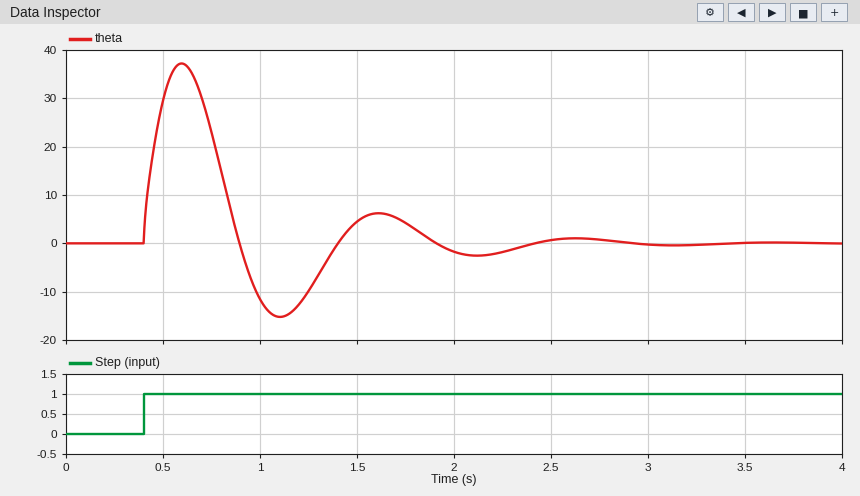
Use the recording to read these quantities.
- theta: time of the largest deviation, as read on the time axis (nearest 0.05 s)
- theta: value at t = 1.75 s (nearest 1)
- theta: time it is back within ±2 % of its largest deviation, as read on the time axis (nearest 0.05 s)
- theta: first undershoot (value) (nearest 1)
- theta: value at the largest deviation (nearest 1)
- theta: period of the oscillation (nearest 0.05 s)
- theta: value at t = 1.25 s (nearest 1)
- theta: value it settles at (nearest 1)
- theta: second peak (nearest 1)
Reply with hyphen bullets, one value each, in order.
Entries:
- 0.60 s
- 4
- 2.75 s
- -15
- 37
- 1.00 s
- -10
- 0
- 6
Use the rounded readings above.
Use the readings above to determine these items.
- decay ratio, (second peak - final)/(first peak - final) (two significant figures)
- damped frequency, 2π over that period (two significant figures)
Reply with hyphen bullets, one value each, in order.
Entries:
- 0.16
- 6.3 rad/s
